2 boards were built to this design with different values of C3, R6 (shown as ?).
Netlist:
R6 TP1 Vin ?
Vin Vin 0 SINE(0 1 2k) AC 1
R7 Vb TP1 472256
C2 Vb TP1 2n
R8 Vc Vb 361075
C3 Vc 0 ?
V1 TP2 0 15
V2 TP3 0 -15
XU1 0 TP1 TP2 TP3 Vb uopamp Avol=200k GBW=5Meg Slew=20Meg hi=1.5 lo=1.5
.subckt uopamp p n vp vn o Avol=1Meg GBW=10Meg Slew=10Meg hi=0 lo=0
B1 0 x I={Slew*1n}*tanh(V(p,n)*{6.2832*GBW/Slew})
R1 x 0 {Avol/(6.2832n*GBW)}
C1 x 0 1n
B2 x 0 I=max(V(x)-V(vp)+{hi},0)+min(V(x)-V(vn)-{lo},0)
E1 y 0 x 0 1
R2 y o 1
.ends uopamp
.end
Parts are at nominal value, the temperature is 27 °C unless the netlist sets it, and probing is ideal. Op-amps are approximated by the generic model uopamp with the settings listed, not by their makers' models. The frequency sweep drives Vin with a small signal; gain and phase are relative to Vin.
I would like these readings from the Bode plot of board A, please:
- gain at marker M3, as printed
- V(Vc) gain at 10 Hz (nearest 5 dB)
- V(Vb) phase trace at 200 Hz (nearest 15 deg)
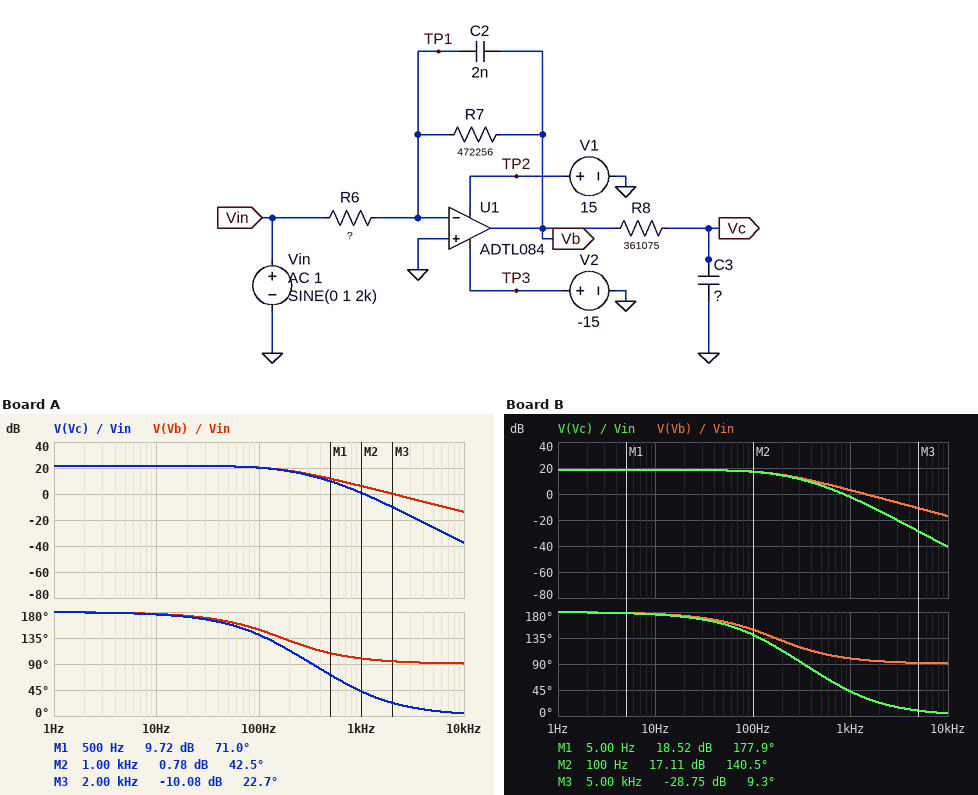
-10.08 dB
20 dB
135 deg
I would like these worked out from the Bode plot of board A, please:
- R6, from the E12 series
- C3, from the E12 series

39 kΩ
680 pF
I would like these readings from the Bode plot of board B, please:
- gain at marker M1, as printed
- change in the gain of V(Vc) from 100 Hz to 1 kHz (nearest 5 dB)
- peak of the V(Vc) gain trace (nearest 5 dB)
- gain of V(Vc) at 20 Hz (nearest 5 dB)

18.52 dB
-20 dB
20 dB
20 dB
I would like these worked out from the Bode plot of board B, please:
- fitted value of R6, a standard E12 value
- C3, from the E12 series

56 kΩ
680 pF
